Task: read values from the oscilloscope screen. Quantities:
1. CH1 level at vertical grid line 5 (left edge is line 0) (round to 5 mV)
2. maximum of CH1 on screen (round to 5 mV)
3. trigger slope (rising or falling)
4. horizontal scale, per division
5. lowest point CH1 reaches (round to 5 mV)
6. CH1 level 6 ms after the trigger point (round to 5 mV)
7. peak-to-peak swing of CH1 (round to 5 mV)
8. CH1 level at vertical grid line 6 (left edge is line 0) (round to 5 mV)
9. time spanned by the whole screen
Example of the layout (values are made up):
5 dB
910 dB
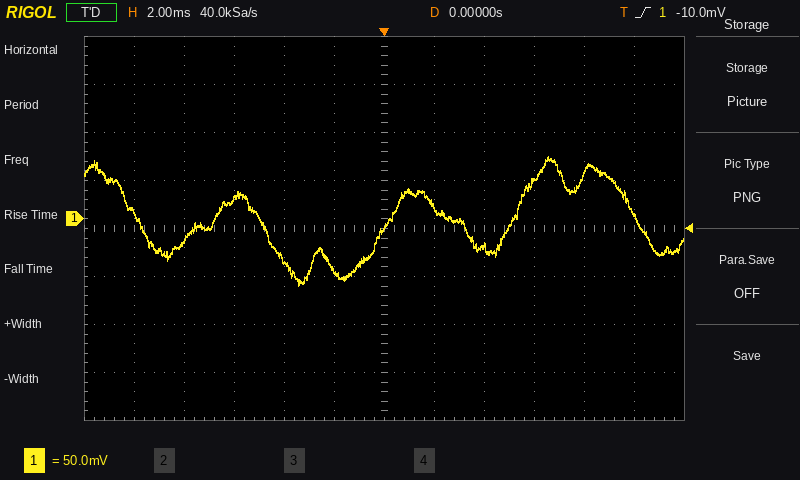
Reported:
-55 mV
65 mV
rising
2 ms
-70 mV
40 mV
135 mV
-10 mV
24 ms
